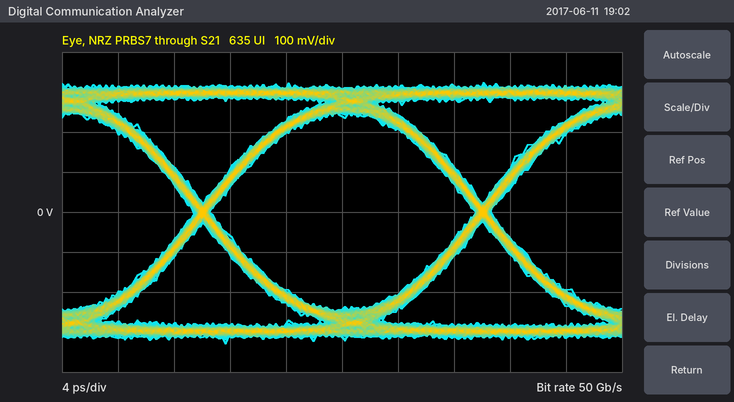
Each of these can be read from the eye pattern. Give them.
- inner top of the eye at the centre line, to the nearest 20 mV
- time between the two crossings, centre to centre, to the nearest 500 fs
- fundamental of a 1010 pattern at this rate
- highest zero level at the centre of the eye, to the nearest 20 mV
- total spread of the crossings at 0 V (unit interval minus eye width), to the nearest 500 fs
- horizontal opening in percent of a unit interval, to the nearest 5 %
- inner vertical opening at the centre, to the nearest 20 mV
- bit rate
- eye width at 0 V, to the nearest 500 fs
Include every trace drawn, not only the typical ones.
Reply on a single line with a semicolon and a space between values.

240 mV; 20.0 ps; 25 GHz; -240 mV; 1.0 ps; 95 %; 480 mV; 50 Gb/s; 19.0 ps
